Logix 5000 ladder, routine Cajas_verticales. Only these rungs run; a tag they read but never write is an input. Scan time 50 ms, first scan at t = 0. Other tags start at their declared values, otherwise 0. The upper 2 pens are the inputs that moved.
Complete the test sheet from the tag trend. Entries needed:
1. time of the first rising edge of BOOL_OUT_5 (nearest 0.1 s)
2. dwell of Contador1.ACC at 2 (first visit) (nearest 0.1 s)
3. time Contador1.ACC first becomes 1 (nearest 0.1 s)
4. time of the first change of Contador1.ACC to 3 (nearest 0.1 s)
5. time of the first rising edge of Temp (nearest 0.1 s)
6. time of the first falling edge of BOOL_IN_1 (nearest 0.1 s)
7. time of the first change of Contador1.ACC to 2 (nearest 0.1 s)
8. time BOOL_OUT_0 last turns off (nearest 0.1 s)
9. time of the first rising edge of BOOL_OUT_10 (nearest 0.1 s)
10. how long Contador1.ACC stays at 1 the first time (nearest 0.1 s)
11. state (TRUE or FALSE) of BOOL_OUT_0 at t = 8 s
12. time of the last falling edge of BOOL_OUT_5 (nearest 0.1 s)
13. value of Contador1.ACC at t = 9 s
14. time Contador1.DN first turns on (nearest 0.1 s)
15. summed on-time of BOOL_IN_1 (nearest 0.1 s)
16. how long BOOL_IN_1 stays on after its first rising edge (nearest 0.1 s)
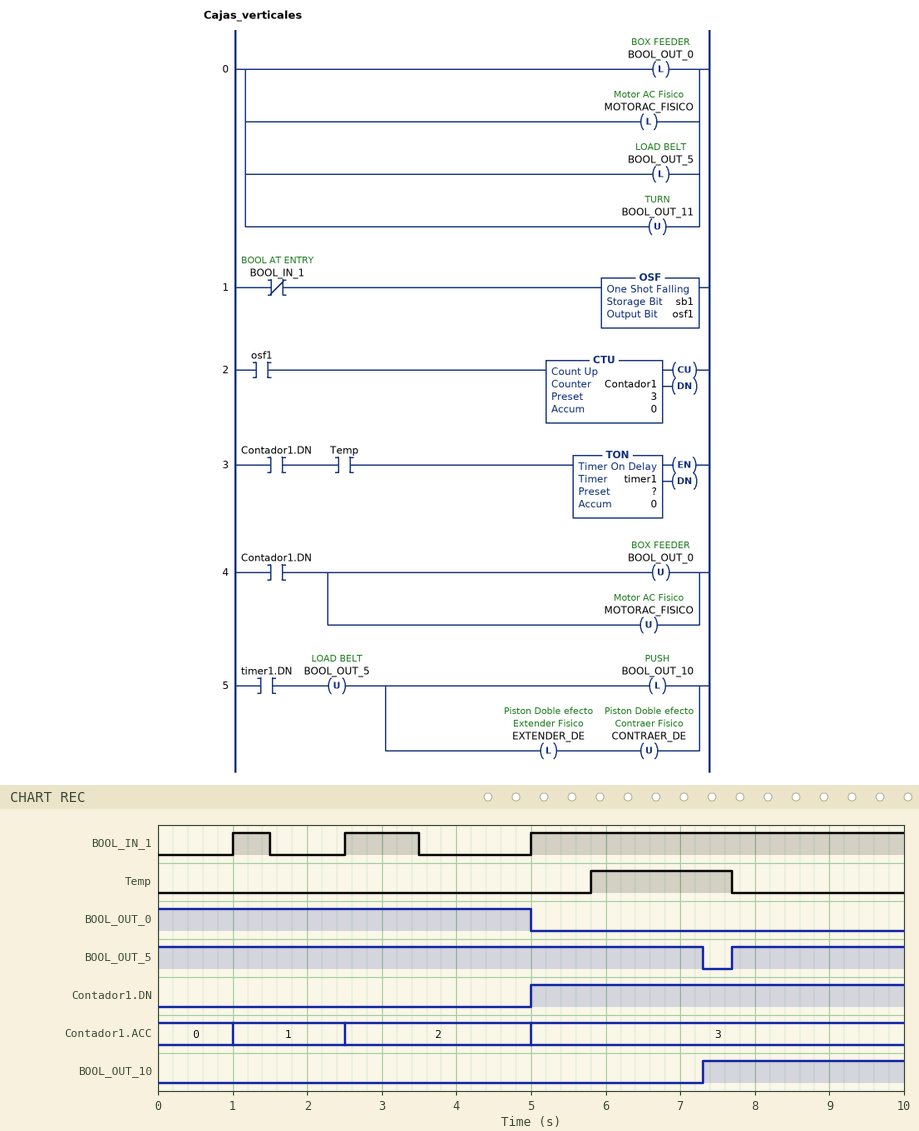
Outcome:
7.7 s
2.5 s
1.0 s
5.0 s
5.8 s
1.5 s
2.5 s
5.0 s
7.3 s
1.5 s
FALSE
7.3 s
3
5.0 s
6.5 s
0.5 s
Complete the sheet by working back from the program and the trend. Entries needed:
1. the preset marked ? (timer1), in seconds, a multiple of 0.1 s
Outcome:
1.5 s
